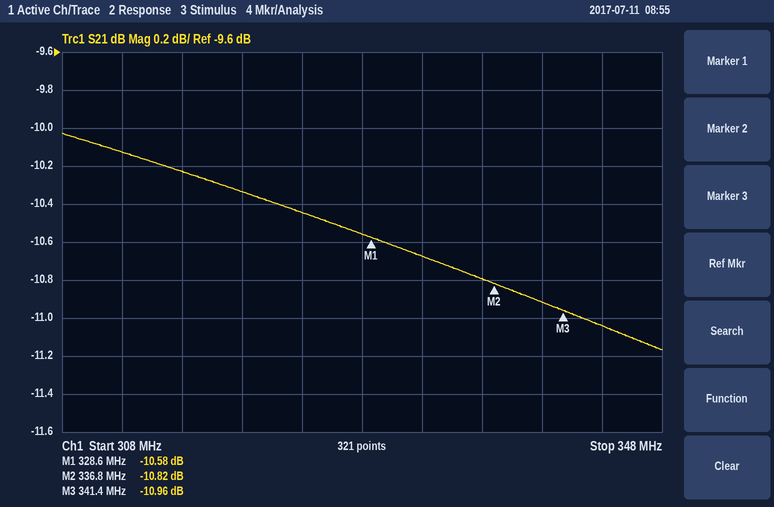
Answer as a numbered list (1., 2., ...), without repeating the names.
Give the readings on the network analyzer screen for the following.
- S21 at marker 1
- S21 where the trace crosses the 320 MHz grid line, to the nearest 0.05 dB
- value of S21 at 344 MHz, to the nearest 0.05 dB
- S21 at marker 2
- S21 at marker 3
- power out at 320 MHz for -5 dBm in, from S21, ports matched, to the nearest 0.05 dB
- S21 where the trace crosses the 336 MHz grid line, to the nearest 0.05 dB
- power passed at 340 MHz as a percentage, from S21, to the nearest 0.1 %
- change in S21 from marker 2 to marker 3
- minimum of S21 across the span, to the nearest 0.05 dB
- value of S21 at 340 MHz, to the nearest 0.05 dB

1. -10.58 dB
2. -10.35 dB
3. -11.05 dB
4. -10.82 dB
5. -10.96 dB
6. -15.35 dBm
7. -10.80 dB
8. 8.1 %
9. -0.14 dB
10. -11.15 dB
11. -10.90 dB
